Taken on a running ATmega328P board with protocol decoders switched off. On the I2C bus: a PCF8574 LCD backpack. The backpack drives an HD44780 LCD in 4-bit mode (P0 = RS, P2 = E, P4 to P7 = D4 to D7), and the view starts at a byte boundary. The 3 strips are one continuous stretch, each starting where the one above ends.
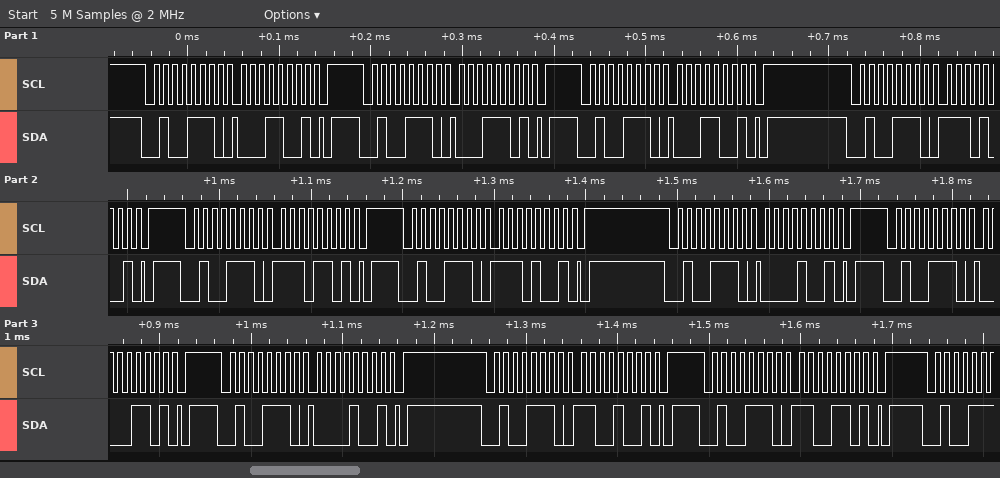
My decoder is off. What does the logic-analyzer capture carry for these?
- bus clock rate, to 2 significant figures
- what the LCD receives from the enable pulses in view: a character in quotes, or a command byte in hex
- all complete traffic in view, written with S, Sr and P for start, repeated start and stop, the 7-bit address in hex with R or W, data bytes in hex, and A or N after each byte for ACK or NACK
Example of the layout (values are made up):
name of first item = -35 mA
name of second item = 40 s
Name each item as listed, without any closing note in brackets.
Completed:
bus clock rate, to 2 significant figures = 100 kHz
what the LCD receives from the enable pulses in view: a character in quotes, or a command byte in hex = data 0x1E
all complete traffic in view, written with S, Sr and P for start, repeated start and stop, the 7-bit address in hex with R or W, data bytes in hex, and A or N after each byte for ACK or NACK = S 27W A 19 A P S 27W A 1D A P S 27W A 19 A P S 27W A E9 A P S 27W A ED A P S 27W A E9 A P S 27W A 09 A P S 27W A 0D A P S 27W A 09 A P S 27W A C9 A P S 27W A CD A P
